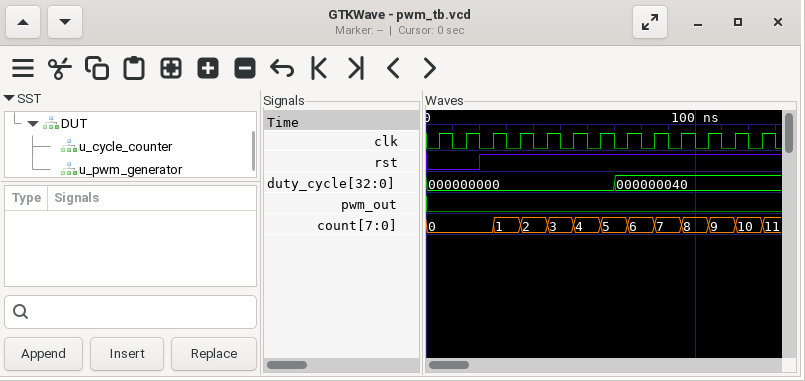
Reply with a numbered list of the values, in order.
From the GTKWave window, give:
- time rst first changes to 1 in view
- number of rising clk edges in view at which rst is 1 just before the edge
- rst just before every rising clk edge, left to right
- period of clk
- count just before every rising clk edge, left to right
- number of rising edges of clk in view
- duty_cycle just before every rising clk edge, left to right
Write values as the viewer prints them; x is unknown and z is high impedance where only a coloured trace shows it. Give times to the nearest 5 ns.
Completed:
1. 20 ns
2. 11
3. 0 0 1 1 1 1 1 1 1 1 1 1 1
4. 10 ns
5. 0, 0, 0, 1, 2, 3, 4, 5, 6, 7, 8, 9, 10
6. 13
7. 000000000, 000000000, 000000000, 000000000, 000000000, 000000000, 000000000, 000000040, 000000040, 000000040, 000000040, 000000040, 000000040
